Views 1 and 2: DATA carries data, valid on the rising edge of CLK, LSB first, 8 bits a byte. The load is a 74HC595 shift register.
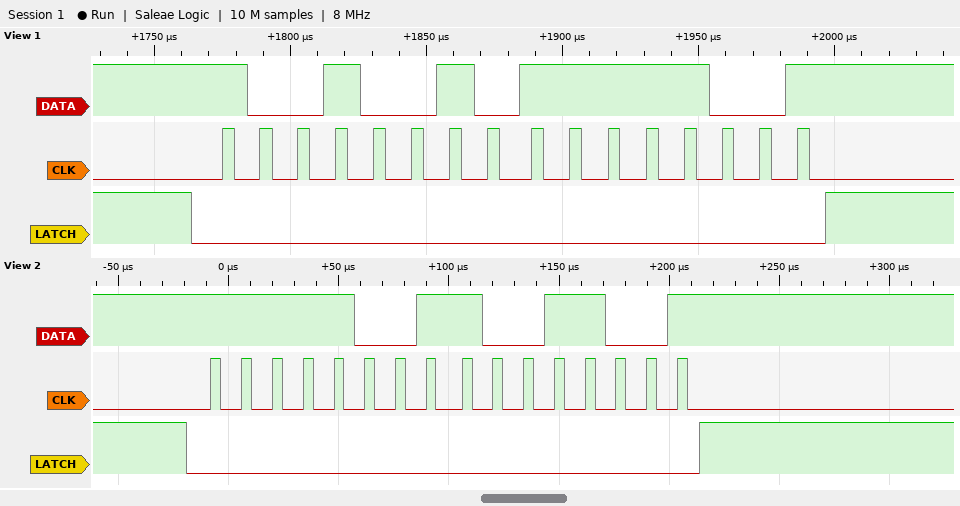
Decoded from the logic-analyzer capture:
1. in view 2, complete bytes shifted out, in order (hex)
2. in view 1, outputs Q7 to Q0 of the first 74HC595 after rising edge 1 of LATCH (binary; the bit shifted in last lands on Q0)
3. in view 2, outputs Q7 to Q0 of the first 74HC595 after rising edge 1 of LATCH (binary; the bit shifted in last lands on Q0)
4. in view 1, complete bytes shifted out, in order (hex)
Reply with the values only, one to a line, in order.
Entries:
9F 99
11111001
10011001
0x49 0x9F
